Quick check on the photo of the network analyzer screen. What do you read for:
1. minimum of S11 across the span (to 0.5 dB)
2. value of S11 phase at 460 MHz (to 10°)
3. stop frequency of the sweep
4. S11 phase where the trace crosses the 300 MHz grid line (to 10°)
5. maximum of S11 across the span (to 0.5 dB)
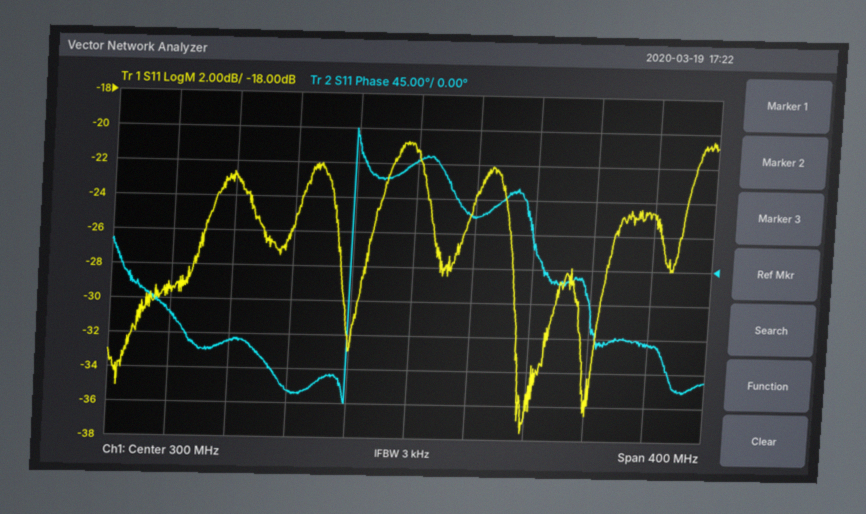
-37.5 dB
-100°
500 MHz
140°
-20.5 dB
